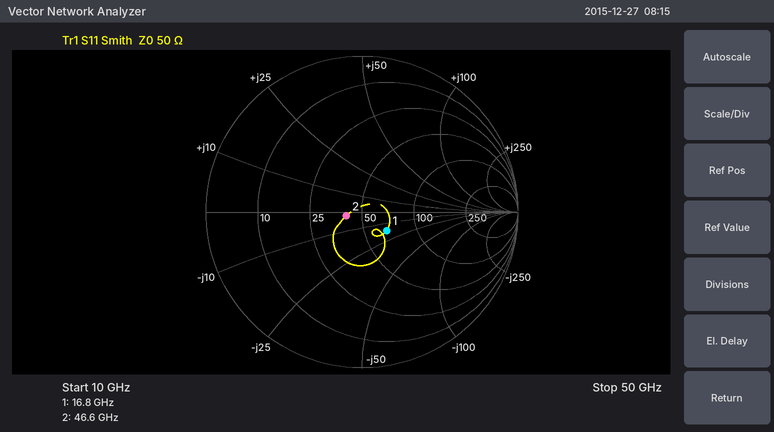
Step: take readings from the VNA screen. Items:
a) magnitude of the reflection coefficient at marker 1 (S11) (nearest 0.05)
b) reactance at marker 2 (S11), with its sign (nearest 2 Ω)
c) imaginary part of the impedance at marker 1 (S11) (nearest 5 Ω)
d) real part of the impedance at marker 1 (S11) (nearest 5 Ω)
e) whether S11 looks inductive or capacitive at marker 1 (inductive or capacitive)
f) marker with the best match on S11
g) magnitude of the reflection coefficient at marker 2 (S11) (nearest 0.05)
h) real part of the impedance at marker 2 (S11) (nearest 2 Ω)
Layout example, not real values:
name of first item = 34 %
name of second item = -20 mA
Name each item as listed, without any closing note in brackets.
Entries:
magnitude of the reflection coefficient at marker 1 (S11) = 0.20
reactance at marker 2 (S11), with its sign = -2 Ω
imaginary part of the impedance at marker 1 (S11) = -15 Ω
real part of the impedance at marker 1 (S11) = 65 Ω
whether S11 looks inductive or capacitive at marker 1 = capacitive
marker with the best match on S11 = marker 2
magnitude of the reflection coefficient at marker 2 (S11) = 0.10
real part of the impedance at marker 2 (S11) = 40 Ω
